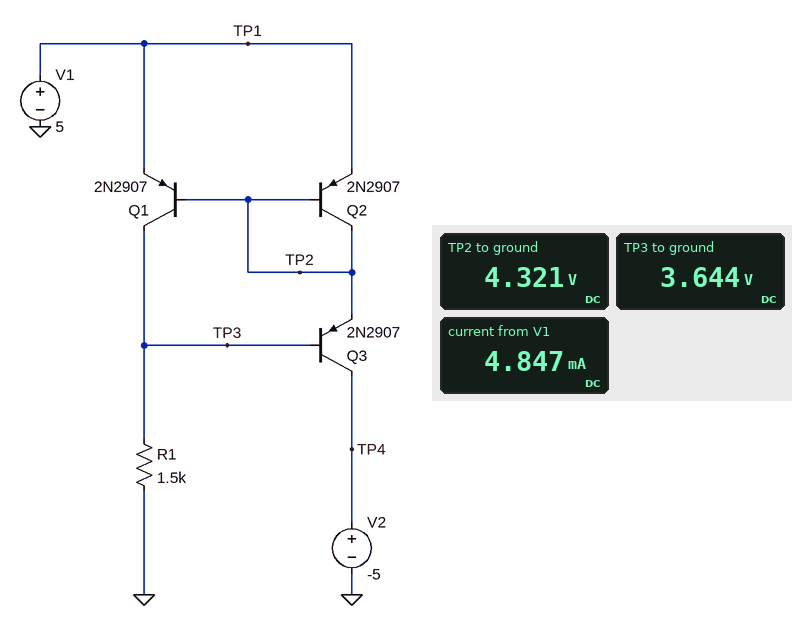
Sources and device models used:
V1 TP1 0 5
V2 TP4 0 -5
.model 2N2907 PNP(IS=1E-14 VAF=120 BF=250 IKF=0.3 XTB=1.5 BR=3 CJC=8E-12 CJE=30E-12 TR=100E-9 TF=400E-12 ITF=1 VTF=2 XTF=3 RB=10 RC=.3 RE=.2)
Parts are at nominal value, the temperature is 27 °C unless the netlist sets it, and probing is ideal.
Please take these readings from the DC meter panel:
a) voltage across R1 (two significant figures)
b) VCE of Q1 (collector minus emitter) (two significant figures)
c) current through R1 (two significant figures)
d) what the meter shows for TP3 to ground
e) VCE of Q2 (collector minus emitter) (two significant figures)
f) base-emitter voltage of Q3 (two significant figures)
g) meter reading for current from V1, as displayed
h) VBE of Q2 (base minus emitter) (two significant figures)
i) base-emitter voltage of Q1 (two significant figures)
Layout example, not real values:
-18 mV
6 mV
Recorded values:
3.6 V
-1.4 V
2.4 mA
3.644 V
-680 mV
-680 mV
4.847 mA
-680 mV
-680 mV
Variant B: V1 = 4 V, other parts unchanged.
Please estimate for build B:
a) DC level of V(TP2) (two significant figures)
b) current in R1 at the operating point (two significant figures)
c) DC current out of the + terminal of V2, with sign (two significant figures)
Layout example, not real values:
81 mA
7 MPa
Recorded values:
3.3 V
1.8 mA
-1.8 mA
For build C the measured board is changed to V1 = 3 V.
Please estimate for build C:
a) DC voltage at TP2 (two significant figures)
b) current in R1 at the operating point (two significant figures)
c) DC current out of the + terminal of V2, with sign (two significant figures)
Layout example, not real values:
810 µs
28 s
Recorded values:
2.3 V
1.1 mA
-1.1 mA
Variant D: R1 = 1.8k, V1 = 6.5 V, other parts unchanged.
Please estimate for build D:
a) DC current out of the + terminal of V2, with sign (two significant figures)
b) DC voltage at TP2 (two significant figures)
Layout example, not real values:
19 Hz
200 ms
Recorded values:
-2.8 mA
5.8 V
